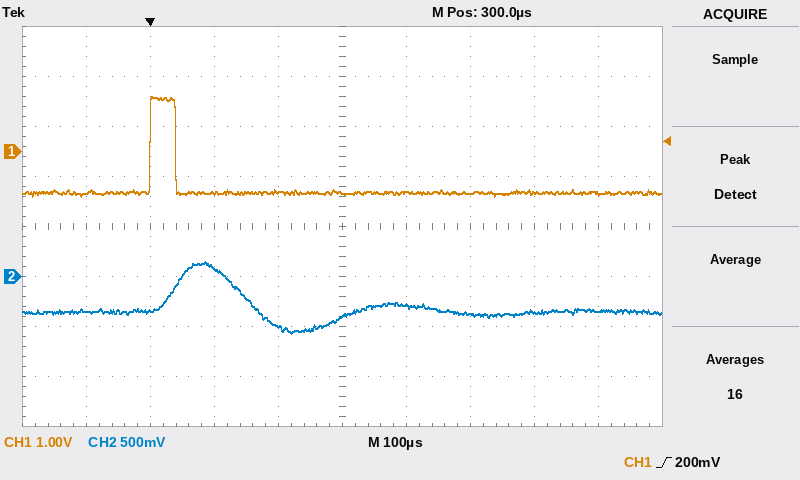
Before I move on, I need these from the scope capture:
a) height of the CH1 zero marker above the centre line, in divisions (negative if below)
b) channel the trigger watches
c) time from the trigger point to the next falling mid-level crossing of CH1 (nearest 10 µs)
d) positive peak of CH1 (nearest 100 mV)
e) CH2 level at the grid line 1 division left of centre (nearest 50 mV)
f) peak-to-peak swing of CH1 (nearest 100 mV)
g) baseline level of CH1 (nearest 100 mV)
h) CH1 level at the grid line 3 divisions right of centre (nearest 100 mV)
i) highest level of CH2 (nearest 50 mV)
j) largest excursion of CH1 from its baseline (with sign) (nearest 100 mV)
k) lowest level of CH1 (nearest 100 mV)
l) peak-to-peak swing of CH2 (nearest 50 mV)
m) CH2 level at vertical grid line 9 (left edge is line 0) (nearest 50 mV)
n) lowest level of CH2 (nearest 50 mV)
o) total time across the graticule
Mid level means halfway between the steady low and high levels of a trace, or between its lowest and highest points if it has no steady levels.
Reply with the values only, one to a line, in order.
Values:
+1.5 div
CH1
40 µs
1.1 V
-500 mV
2.0 V
-800 mV
-800 mV
150 mV
+1.9 V
-900 mV
700 mV
-350 mV
-550 mV
1 ms
